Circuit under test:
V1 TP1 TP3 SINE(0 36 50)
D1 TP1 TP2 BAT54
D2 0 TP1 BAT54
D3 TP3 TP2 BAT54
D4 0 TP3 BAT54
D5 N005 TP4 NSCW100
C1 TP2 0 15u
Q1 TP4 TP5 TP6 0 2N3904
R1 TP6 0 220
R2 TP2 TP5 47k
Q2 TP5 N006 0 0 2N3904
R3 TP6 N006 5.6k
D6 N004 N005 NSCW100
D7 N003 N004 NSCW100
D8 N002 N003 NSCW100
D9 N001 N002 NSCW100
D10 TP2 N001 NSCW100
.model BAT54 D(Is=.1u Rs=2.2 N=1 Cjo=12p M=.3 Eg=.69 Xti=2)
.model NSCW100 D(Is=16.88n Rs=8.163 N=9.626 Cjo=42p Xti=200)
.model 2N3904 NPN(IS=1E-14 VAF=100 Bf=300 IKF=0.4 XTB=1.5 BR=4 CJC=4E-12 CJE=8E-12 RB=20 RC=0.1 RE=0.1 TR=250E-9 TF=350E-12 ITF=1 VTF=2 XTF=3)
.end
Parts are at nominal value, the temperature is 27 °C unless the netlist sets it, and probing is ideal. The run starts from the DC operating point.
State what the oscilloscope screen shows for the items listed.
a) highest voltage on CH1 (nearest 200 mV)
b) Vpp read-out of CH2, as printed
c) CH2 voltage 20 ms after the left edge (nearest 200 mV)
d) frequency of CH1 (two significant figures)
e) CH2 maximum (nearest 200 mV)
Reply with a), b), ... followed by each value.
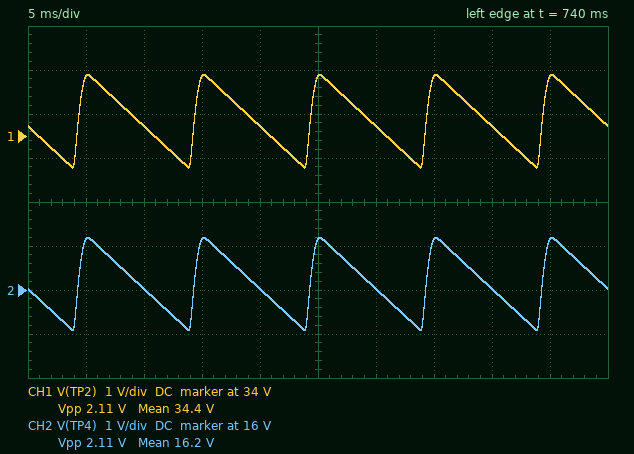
a) 35.4 V
b) 2.11 V
c) 16.0 V
d) 100 Hz
e) 17.2 V
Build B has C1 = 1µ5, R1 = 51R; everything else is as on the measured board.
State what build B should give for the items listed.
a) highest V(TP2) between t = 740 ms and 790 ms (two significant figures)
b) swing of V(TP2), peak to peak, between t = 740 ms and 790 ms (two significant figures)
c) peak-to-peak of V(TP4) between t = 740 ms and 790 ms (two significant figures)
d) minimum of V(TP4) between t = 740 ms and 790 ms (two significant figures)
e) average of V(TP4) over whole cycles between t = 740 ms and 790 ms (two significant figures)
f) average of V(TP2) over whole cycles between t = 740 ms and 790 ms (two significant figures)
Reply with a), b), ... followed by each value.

a) 35 V
b) 20 V
c) 14 V
d) 57 mV
e) 5.7 V
f) 25 V
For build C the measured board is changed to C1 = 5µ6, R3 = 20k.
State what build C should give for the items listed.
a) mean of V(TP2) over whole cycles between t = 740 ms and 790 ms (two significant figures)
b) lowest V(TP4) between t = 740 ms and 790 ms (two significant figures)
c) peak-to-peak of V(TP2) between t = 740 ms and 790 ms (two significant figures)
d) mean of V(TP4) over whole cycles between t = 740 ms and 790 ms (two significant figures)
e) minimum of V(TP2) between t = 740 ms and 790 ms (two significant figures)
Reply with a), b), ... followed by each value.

a) 33 V
b) 12 V
c) 5.4 V
d) 15 V
e) 30 V
